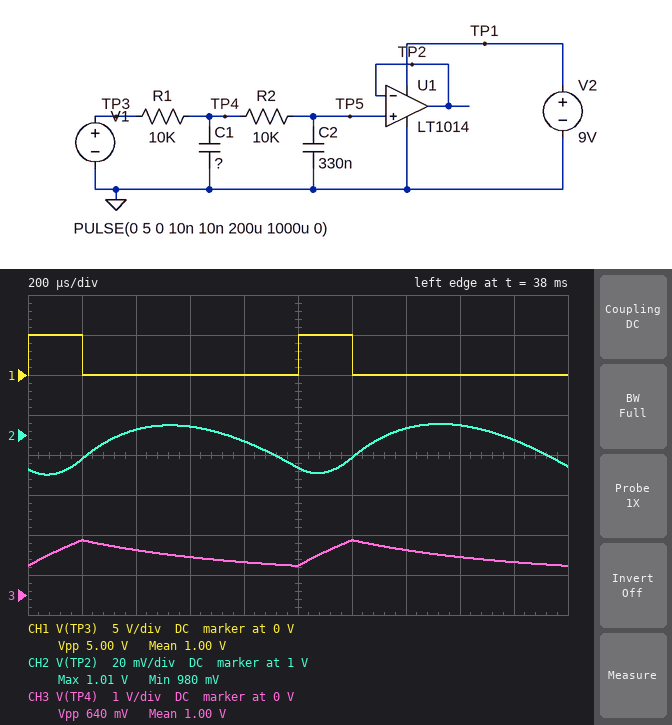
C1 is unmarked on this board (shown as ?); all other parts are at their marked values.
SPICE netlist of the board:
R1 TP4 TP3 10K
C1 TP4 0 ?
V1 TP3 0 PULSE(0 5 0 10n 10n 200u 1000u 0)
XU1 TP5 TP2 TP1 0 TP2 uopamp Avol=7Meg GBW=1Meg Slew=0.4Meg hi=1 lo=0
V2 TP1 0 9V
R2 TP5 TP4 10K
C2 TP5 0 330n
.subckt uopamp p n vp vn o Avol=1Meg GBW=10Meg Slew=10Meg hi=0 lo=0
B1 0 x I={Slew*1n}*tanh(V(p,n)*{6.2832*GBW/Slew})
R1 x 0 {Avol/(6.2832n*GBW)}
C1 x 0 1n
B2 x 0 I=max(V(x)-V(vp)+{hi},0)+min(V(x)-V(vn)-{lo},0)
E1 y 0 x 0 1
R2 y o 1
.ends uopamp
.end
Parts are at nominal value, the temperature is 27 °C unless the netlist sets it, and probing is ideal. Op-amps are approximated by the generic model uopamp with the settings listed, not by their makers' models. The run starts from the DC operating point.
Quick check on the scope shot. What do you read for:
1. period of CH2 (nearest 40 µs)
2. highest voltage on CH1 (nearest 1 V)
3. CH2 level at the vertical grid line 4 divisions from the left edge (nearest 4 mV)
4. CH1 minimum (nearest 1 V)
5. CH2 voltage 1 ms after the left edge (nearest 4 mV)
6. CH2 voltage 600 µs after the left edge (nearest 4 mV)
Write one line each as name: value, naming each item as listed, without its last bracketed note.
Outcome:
period of CH2: 1.00 ms
highest voltage on CH1: 5 V
CH2 level at the vertical grid line 4 divisions from the left edge: 996 mV
CH1 minimum: 0 V
CH2 voltage 1 ms after the left edge: 984 mV
CH2 voltage 600 µs after the left edge: 1.004 V
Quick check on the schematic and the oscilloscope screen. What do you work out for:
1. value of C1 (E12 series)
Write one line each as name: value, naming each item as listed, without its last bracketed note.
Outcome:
value of C1: 120 nF
